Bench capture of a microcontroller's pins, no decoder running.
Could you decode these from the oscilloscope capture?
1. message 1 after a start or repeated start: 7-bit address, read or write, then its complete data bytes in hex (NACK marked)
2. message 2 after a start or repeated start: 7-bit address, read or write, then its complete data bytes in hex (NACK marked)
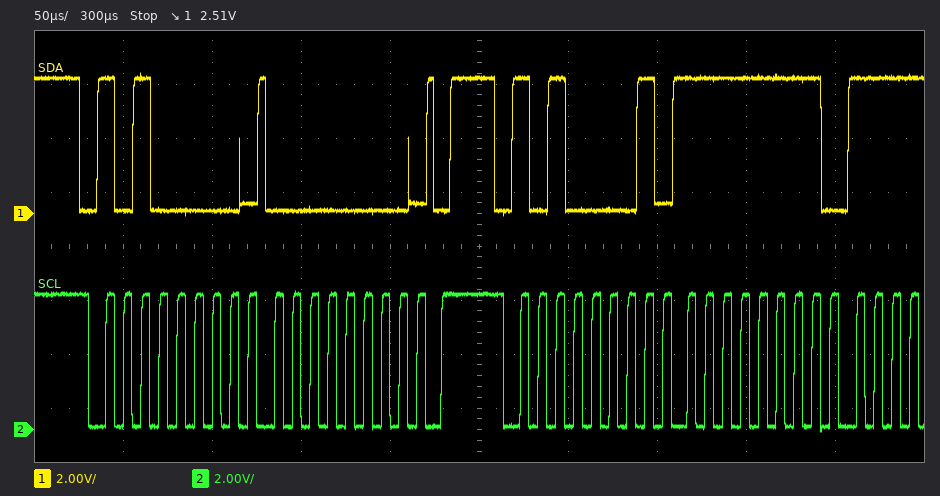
0x50 write: 00
0x50 read: FF
